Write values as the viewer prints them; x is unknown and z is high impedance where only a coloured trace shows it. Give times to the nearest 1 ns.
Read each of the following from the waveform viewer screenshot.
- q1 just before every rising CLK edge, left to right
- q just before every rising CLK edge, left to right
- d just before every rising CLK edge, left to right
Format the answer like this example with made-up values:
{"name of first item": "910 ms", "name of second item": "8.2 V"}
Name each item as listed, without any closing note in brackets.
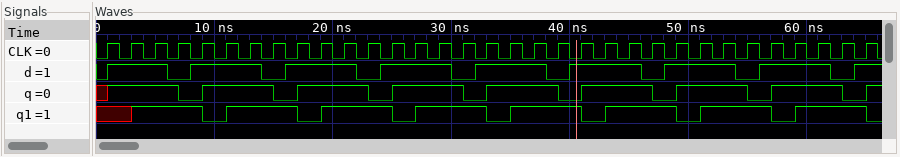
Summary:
{"q1 just before every rising CLK edge, left to right": "x x 1 1 1 0 1 1 1 0 1 1 1 0 1 1 1 0 1 1 1 0 1 1 1 0 1 1 1 0 1 1 1", "q just before every rising CLK edge, left to right": "x 1 1 1 0 1 1 1 0 1 1 1 0 1 1 1 0 1 1 1 0 1 1 1 0 1 1 1 0 1 1 1 0", "d just before every rising CLK edge, left to right": "0 1 1 0 1 1 1 0 1 1 1 0 1 1 1 0 1 1 1 0 1 1 1 0 1 1 1 0 1 1 1 0 1"}
